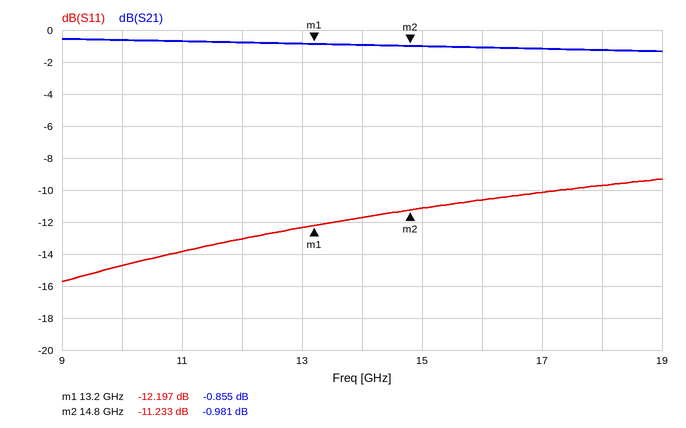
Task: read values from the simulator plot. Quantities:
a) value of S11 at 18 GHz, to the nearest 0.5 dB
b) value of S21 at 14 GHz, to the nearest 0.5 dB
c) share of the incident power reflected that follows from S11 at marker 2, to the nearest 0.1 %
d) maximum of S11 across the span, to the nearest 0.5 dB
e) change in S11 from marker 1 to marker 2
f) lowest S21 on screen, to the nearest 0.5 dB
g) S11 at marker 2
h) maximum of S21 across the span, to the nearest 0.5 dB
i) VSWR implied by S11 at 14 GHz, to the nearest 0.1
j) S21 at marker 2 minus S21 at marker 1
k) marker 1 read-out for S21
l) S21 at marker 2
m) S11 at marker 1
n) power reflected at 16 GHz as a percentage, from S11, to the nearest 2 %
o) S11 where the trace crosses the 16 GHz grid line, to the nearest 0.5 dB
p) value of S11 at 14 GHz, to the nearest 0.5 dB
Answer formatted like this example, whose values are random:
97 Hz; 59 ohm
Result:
-9.5 dB; -1.0 dB; 7.5 %; -9.5 dB; 0.964 dB; -1.5 dB; -11.233 dB; -0.5 dB; 1.7; -0.126 dB; -0.855 dB; -0.981 dB; -12.197 dB; 8 %; -10.5 dB; -11.5 dB
